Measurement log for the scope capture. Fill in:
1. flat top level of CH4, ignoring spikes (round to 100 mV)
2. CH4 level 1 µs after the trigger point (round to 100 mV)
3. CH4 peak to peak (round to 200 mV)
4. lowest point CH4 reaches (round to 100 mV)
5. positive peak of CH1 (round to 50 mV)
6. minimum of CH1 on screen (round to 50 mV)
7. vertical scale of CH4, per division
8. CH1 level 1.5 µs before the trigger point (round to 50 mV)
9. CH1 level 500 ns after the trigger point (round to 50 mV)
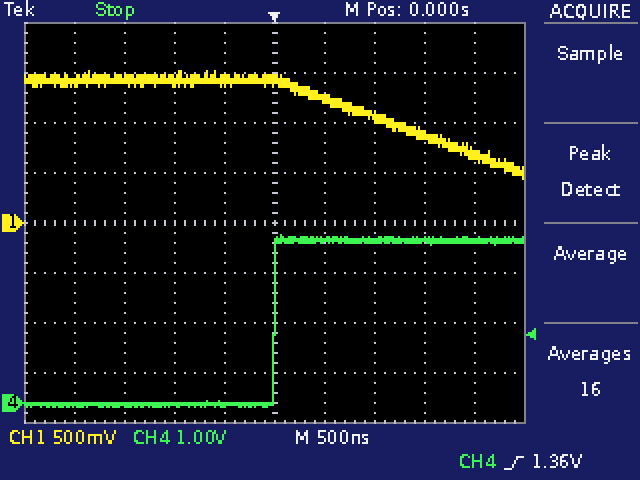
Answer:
3.2 V
3.2 V
3.4 V
-100 mV
1.50 V
450 mV
1 V
1.45 V
1.25 V
